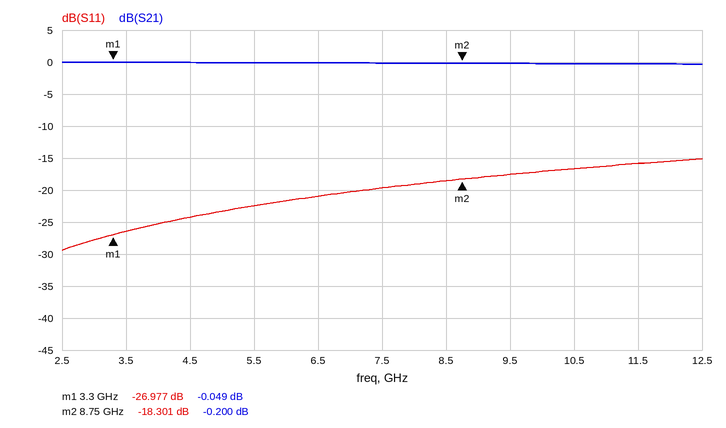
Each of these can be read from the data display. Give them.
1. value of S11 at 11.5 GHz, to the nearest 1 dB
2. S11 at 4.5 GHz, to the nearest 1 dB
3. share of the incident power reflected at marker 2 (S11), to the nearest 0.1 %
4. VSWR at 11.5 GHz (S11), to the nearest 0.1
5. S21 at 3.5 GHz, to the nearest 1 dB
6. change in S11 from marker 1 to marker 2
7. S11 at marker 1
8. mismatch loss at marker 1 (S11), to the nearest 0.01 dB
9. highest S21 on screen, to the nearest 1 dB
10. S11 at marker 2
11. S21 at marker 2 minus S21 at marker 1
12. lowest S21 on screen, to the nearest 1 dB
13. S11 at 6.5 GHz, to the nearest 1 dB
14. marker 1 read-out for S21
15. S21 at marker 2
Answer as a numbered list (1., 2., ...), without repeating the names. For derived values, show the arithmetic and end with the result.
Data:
1. -16 dB
2. -24 dB
3. 10^(-18.301/10) ≈ 1.5 %
4. |Γ| = 10^(-16/20) = 0.1585; VSWR = (1 + 0.1585)/(1 − 0.1585) ≈ 1.4
5. 0 dB
6. -18.301 − (-26.977) = 8.676 dB
7. -26.977 dB
8. −10 log10(1 − 10^(-26.977/10)) ≈ 0.01 dB
9. 0 dB
10. -18.301 dB
11. -0.2 − (-0.049) = -0.151 dB
12. 0 dB
13. -21 dB
14. -0.049 dB
15. -0.200 dB
